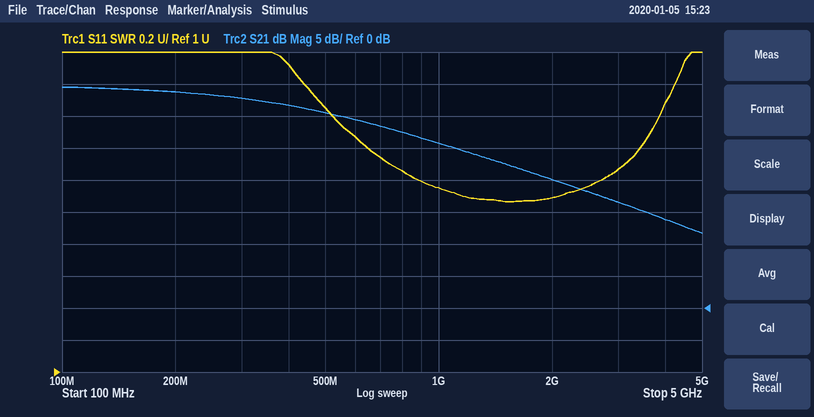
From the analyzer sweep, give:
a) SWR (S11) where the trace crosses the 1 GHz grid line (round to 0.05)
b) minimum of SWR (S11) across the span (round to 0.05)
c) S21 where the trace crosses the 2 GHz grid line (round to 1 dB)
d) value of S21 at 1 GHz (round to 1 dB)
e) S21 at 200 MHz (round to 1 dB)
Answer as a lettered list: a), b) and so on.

a) 2.15
b) 2.05
c) 20 dB
d) 26 dB
e) 34 dB
